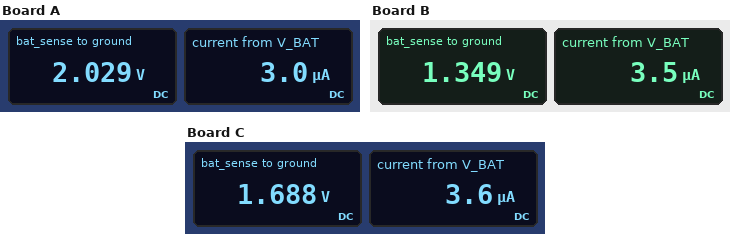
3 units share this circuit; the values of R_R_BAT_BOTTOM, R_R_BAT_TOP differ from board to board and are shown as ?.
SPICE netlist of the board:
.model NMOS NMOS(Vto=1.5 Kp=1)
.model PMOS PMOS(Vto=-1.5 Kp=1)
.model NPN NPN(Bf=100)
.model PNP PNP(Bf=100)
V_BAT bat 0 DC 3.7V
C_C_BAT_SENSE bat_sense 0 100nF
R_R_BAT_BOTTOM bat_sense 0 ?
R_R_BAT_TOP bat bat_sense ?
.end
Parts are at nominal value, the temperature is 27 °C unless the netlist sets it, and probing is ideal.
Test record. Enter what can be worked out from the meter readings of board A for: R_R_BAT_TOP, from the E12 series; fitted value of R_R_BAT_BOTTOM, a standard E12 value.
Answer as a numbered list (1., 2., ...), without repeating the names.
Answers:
1. 560 kΩ
2. 680 kΩ
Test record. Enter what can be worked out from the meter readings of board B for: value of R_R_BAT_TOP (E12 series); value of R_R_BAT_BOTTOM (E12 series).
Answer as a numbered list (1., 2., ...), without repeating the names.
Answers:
1. 680 kΩ
2. 390 kΩ
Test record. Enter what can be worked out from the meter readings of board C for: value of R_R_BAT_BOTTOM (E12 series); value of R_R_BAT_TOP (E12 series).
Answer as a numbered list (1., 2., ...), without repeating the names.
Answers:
1. 470 kΩ
2. 560 kΩ
